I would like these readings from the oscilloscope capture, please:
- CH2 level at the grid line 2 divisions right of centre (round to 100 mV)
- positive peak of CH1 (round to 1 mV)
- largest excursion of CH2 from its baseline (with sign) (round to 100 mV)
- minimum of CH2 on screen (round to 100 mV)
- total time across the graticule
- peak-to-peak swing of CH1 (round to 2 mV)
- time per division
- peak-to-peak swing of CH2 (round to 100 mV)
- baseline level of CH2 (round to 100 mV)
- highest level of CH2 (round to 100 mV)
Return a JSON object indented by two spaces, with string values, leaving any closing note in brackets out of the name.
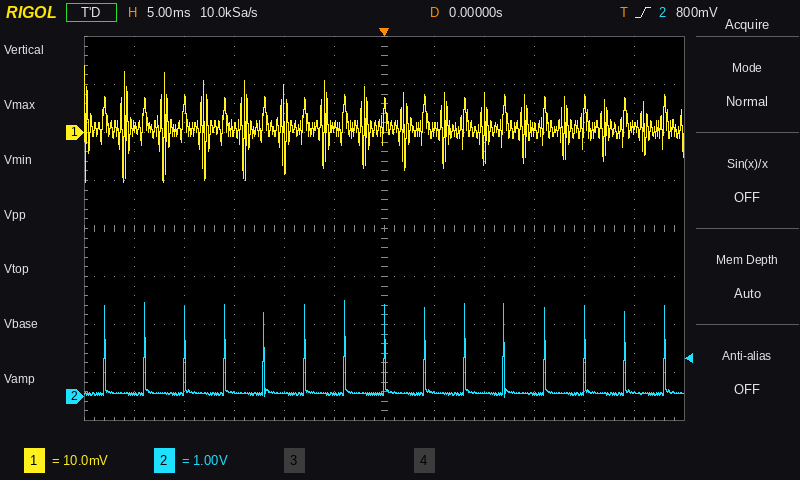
{
  "CH2 level at the grid line 2 divisions right of centre": "100 mV",
  "positive peak of CH1": "14 mV",
  "largest excursion of CH2 from its baseline (with sign)": "+1.9 V",
  "minimum of CH2 on screen": "0.0 V",
  "total time across the graticule": "60 ms",
  "peak-to-peak swing of CH1": "24 mV",
  "time per division": "5 ms",
  "peak-to-peak swing of CH2": "2.0 V",
  "baseline level of CH2": "100 mV",
  "highest level of CH2": "2.0 V"
}
